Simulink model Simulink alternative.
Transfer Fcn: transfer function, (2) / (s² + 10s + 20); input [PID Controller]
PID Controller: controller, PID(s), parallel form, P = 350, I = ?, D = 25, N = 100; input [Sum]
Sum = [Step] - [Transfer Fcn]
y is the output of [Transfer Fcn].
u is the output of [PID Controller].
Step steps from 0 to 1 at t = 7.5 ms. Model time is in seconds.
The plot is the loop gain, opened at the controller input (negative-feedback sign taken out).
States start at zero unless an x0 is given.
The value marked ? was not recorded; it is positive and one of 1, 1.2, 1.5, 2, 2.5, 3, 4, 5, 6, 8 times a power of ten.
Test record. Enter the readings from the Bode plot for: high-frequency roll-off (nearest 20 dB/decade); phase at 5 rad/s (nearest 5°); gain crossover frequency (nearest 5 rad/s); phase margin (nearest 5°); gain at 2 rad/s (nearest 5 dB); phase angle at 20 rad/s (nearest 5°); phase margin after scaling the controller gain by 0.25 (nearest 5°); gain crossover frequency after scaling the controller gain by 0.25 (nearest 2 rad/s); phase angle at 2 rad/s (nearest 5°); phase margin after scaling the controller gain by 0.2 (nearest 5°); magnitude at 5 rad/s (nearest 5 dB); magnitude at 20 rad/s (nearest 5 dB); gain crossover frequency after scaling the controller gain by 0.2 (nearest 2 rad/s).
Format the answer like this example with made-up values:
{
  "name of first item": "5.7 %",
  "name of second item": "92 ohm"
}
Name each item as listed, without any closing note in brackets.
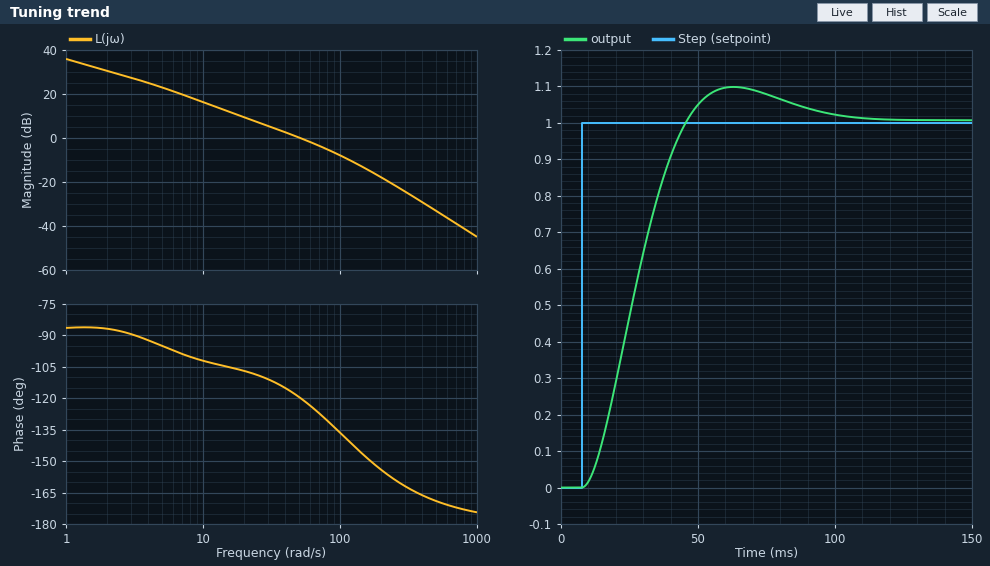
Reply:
{
  "high-frequency roll-off": "-40 dB/decade",
  "phase at 5 rad/s": "-95°",
  "gain crossover frequency": "50 rad/s",
  "phase margin": "60°",
  "gain at 2 rad/s": "30 dB",
  "phase angle at 20 rad/s": "-105°",
  "phase margin after scaling the controller gain by 0.25": "75°",
  "gain crossover frequency after scaling the controller gain by 0.25": "16 rad/s",
  "phase angle at 2 rad/s": "-85°",
  "phase margin after scaling the controller gain by 0.2": "75°",
  "magnitude at 5 rad/s": "25 dB",
  "magnitude at 20 rad/s": "10 dB",
  "gain crossover frequency after scaling the controller gain by 0.2": "12 rad/s"
}
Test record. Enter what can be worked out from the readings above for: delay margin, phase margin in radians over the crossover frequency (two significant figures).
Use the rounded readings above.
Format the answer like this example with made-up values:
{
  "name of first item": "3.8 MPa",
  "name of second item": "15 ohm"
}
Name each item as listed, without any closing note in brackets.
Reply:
{
  "delay margin, phase margin in radians over the crossover frequency": "0.021 s"
}
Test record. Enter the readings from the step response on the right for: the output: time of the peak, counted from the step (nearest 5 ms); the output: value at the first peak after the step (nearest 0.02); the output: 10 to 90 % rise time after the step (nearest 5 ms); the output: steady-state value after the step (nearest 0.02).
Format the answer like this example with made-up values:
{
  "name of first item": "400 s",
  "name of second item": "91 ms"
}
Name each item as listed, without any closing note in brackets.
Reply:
{
  "the output: time of the peak, counted from the step": "55 ms",
  "the output: value at the first peak after the step": "1.10",
  "the output: 10 to 90 % rise time after the step": "25 ms",
  "the output: steady-state value after the step": "1.00"
}
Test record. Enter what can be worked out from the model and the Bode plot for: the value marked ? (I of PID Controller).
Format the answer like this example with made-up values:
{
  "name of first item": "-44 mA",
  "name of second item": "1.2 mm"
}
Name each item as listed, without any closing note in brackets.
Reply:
{
  "the value marked ?": "600"
}
